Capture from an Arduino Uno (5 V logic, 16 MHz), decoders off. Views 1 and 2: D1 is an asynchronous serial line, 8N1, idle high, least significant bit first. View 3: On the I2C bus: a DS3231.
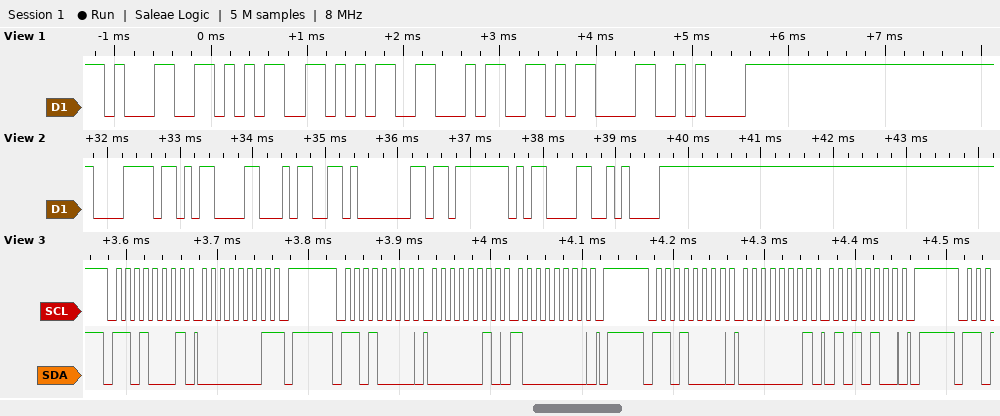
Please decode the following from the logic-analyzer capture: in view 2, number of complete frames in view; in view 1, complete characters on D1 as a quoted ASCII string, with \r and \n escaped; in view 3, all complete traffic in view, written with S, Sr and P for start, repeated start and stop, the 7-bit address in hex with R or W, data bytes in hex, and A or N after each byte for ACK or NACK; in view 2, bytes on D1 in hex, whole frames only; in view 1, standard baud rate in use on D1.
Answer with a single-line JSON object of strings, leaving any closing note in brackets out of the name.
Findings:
{"in view 2, number of complete frames in view": "7", "in view 1, complete characters on D1 as a quoted ASCII string, with \\r and \\n escaped": "\"1554\\r\\n\"", "in view 3, all complete traffic in view, written with S, Sr and P for start, repeated start and stop, the 7-bit address in hex with R or W, data bytes in hex, and A or N after each byte for ACK or NACK": "S 68R A 01 N P S 68W A 02 A 80 A P S 68W A 01 A 54 A P", "in view 2, bytes on D1 in hex, whole frames only": "78 0D 34 01 FB 0D 0A", "in view 1, standard baud rate in use on D1": "9600 baud"}
